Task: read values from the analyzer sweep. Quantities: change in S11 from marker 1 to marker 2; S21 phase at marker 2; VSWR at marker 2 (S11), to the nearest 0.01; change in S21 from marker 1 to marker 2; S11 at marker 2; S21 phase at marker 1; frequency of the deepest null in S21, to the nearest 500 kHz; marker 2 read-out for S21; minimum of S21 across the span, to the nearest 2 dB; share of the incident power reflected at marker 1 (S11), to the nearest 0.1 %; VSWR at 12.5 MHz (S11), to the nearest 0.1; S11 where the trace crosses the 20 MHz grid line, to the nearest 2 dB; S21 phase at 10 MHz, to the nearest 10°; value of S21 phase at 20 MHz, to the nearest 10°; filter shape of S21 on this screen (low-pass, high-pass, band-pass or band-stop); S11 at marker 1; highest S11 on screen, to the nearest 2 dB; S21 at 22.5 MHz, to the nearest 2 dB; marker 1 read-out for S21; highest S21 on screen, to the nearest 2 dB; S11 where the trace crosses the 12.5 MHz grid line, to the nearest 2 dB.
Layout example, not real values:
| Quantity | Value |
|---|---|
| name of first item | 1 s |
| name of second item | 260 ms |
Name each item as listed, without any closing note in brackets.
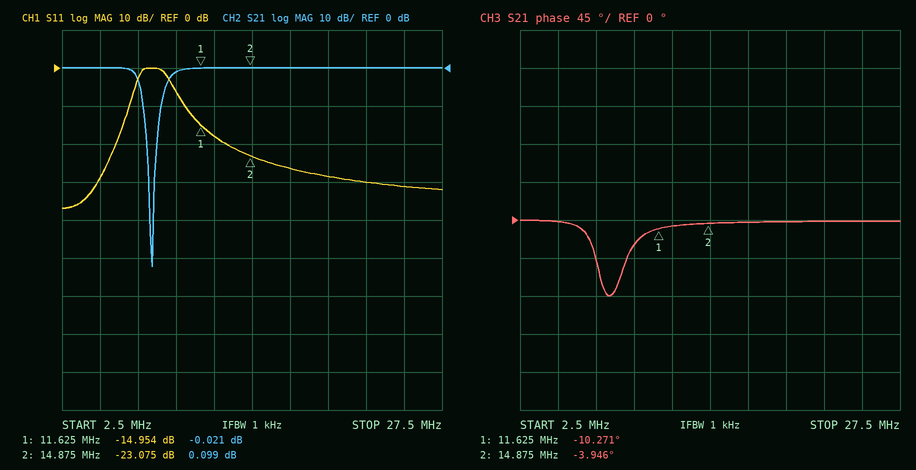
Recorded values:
| Quantity | Value |
|---|---|
| change in S11 from marker 1 to marker 2 | -8.121 dB |
| S21 phase at marker 2 | -3.946° |
| VSWR at marker 2 (S11), to the nearest 0.01 | 1.15 |
| change in S21 from marker 1 to marker 2 | 0.120 dB |
| S11 at marker 2 | -23.075 dB |
| S21 phase at marker 1 | -10.271° |
| frequency of the deepest null in S21, to the nearest 500 kHz | 8.5 MHz |
| marker 2 read-out for S21 | 0.099 dB |
| minimum of S21 across the span, to the nearest 2 dB | -52 dB |
| share of the incident power reflected at marker 1 (S11), to the nearest 0.1 % | 3.2 % |
| VSWR at 12.5 MHz (S11), to the nearest 0.1 | 1.3 |
| S11 where the trace crosses the 20 MHz grid line, to the nearest 2 dB | -28 dB |
| S21 phase at 10 MHz, to the nearest 10° | -30° |
| value of S21 phase at 20 MHz, to the nearest 10° | 0° |
| filter shape of S21 on this screen | band-stop |
| S11 at marker 1 | -14.954 dB |
| highest S11 on screen, to the nearest 2 dB | 0 dB |
| S21 at 22.5 MHz, to the nearest 2 dB | 0 dB |
| marker 1 read-out for S21 | -0.021 dB |
| highest S21 on screen, to the nearest 2 dB | 0 dB |
| S11 where the trace crosses the 12.5 MHz grid line, to the nearest 2 dB | -18 dB |
